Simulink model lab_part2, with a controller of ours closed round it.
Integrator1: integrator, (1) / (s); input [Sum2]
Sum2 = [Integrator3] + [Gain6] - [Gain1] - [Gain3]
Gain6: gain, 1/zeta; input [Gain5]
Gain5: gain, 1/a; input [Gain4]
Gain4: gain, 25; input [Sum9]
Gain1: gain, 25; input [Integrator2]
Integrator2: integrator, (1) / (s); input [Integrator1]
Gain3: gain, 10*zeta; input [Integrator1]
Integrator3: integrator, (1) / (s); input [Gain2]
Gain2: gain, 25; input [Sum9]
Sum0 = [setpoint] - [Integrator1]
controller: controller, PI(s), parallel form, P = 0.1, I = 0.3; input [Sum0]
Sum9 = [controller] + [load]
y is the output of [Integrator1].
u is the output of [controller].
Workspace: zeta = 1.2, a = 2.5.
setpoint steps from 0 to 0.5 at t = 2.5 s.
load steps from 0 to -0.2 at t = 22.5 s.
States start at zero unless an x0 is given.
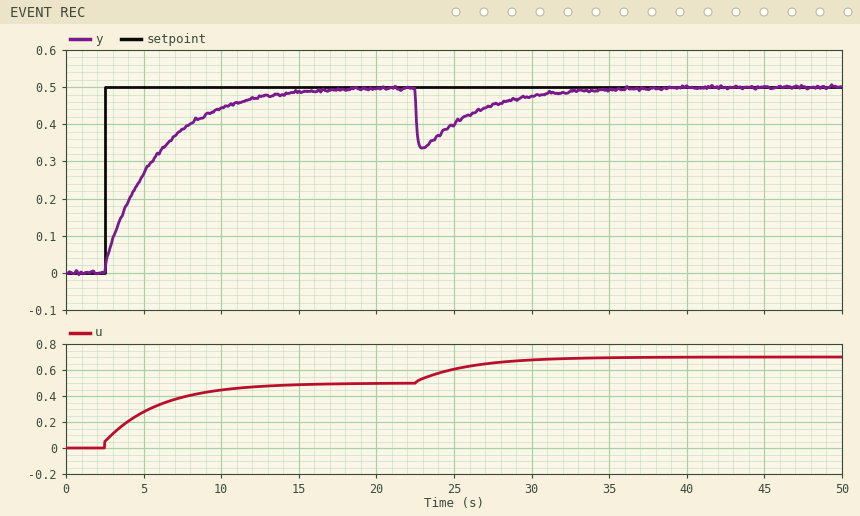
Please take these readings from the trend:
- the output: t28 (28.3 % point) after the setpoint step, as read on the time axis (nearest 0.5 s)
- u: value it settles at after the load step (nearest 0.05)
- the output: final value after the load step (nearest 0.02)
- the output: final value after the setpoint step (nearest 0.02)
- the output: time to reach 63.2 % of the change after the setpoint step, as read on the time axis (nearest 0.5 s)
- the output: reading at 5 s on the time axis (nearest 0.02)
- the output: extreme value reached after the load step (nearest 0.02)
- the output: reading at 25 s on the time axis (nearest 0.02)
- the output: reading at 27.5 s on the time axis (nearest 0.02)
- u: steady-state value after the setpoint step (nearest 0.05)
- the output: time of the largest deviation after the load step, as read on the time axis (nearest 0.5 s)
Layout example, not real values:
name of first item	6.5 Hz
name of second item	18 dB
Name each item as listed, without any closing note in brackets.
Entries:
the output: t28 (28.3 % point) after the setpoint step, as read on the time axis	3.5 s
u: value it settles at after the load step	0.70
the output: final value after the load step	0.50
the output: final value after the setpoint step	0.50
the output: time to reach 63.2 % of the change after the setpoint step, as read on the time axis	6.0 s
the output: reading at 5 s on the time axis	0.26
the output: extreme value reached after the load step	0.34
the output: reading at 25 s on the time axis	0.40
the output: reading at 27.5 s on the time axis	0.46
u: steady-state value after the setpoint step	0.50
the output: time of the largest deviation after the load step, as read on the time axis	23.0 s
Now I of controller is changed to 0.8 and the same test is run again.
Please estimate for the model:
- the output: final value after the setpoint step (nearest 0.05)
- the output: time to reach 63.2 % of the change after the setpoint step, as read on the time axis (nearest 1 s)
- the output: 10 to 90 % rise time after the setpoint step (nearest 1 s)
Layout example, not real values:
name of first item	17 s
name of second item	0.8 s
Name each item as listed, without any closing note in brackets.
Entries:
the output: final value after the setpoint step	0.50
the output: time to reach 63.2 % of the change after the setpoint step, as read on the time axis	4 s
the output: 10 to 90 % rise time after the setpoint step	3 s
